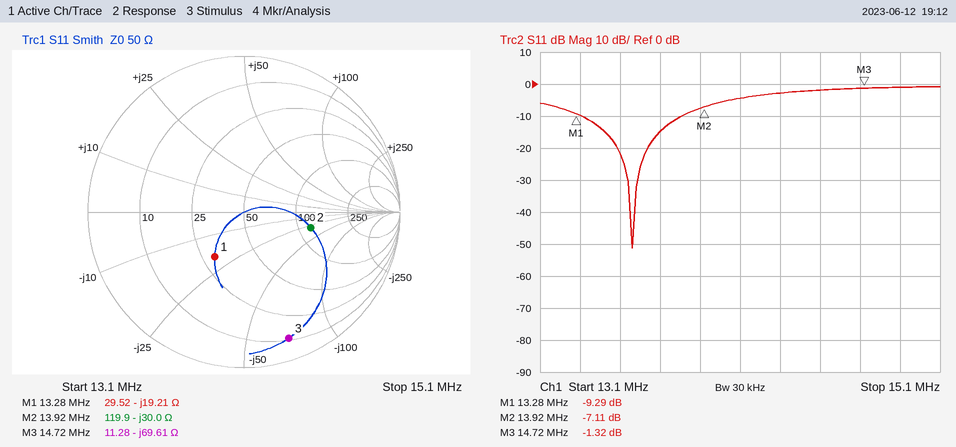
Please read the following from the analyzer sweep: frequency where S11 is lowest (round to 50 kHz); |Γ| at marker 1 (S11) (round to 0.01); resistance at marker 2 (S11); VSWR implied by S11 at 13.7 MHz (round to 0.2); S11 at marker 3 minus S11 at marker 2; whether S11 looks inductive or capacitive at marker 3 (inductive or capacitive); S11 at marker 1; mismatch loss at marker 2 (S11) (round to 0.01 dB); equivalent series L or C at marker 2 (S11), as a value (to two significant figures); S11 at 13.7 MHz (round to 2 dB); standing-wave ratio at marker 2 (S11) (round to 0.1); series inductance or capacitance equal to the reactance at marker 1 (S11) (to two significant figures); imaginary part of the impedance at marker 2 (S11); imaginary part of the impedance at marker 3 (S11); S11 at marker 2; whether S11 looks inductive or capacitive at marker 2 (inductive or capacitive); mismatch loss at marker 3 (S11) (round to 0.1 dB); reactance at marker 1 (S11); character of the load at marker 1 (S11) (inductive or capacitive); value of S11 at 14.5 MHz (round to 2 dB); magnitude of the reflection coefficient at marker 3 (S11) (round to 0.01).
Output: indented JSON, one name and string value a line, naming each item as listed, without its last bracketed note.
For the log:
{
  "frequency where S11 is lowest": "13.55 MHz",
  "|Γ| at marker 1 (S11)": "0.34",
  "resistance at marker 2": "119.9 Ω",
  "VSWR implied by S11 at 13.7 MHz": "1.4",
  "S11 at marker 3 minus S11 at marker 2": "5.79 dB",
  "whether S11 looks inductive or capacitive at marker 3": "capacitive",
  "S11 at marker 1": "-9.29 dB",
  "mismatch loss at marker 2 (S11)": "0.94 dB",
  "equivalent series L or C at marker 2 (S11), as a value": "380 pF",
  "S11 at 13.7 MHz": "-14 dB",
  "standing-wave ratio at marker 2 (S11)": "2.6",
  "series inductance or capacitance equal to the reactance at marker 1 (S11)": "620 pF",
  "imaginary part of the impedance at marker 2": "-30.0 Ω",
  "imaginary part of the impedance at marker 3": "-69.61 Ω",
  "S11 at marker 2": "-7.11 dB",
  "whether S11 looks inductive or capacitive at marker 2": "capacitive",
  "mismatch loss at marker 3 (S11)": "5.8 dB",
  "reactance at marker 1": "-19.21 Ω",
  "character of the load at marker 1 (S11)": "capacitive",
  "value of S11 at 14.5 MHz": "-2 dB",
  "magnitude of the reflection coefficient at marker 3 (S11)": "0.86"
}
